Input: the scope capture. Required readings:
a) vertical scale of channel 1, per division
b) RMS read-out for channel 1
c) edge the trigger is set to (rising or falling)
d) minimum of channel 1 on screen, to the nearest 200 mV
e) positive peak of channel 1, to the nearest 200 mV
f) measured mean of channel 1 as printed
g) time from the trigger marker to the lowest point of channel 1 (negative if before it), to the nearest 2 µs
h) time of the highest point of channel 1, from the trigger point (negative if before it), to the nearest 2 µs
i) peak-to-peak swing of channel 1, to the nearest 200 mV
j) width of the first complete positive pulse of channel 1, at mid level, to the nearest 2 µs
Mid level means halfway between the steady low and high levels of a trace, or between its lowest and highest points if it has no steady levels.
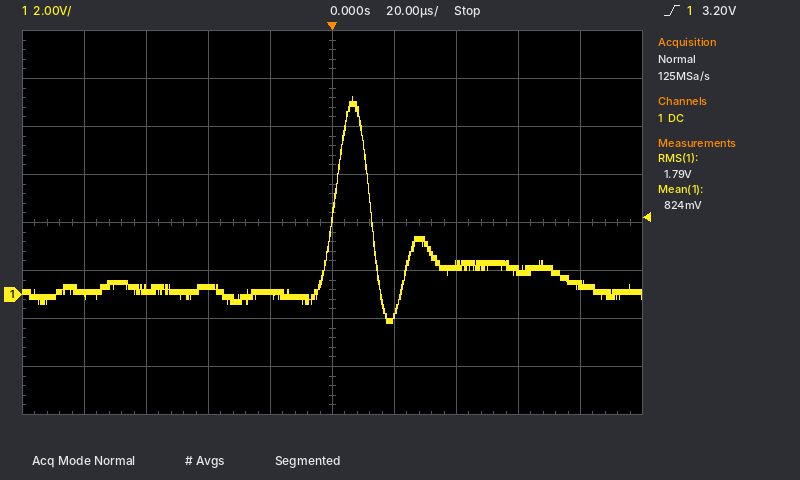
2 V
1.79 V
rising
-1.2 V
8.2 V
824 mV
+18 µs
+6 µs
9.4 V
12 µs
